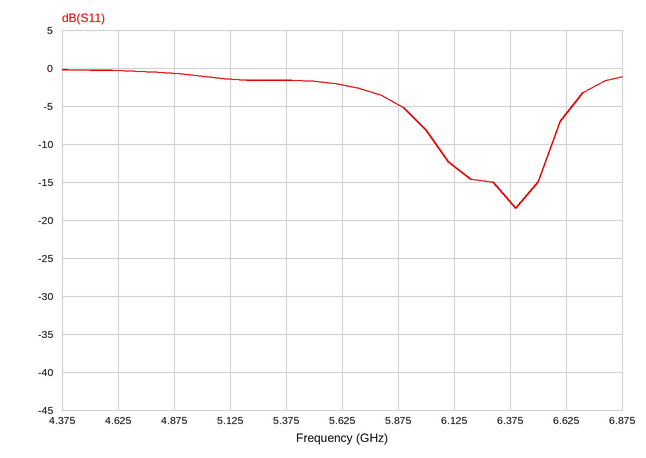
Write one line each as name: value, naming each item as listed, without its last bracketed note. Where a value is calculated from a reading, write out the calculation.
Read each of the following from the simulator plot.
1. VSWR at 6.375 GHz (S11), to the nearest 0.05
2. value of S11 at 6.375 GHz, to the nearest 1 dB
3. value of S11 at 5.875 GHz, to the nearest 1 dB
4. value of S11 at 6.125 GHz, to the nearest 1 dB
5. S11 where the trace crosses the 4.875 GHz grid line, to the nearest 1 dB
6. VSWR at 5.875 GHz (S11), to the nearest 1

VSWR at 6.375 GHz (S11), to the nearest 0.05: |Γ| = 10^(-18/20) = 0.1259; VSWR = (1 + 0.1259)/(1 − 0.1259) ≈ 1.29, so 1.30 to the nearest 0.05
value of S11 at 6.375 GHz, to the nearest 1 dB: -18 dB
value of S11 at 5.875 GHz, to the nearest 1 dB: -5 dB
value of S11 at 6.125 GHz, to the nearest 1 dB: -13 dB
S11 where the trace crosses the 4.875 GHz grid line, to the nearest 1 dB: -1 dB
VSWR at 5.875 GHz (S11), to the nearest 1: |Γ| = 10^(-5/20) = 0.5623; VSWR = (1 + 0.5623)/(1 − 0.5623) ≈ 4
